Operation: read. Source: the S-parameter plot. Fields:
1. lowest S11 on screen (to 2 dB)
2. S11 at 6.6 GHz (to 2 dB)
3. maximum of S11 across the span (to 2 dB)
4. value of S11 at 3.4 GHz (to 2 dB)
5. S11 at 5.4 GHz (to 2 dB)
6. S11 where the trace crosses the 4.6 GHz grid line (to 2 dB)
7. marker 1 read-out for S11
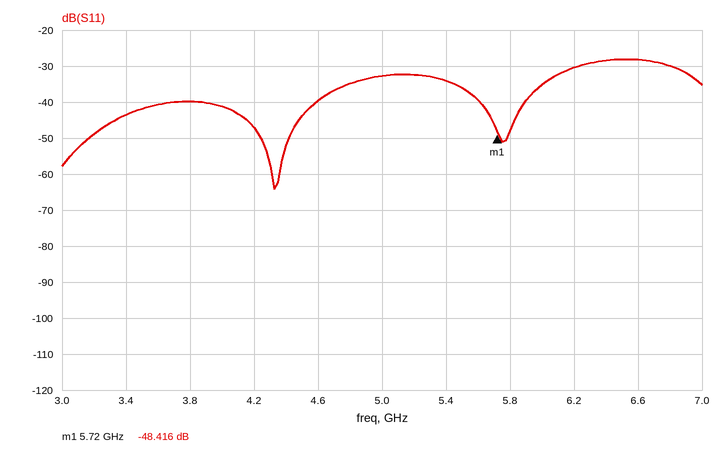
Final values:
-64 dB
-28 dB
-28 dB
-44 dB
-34 dB
-40 dB
-48.416 dB
